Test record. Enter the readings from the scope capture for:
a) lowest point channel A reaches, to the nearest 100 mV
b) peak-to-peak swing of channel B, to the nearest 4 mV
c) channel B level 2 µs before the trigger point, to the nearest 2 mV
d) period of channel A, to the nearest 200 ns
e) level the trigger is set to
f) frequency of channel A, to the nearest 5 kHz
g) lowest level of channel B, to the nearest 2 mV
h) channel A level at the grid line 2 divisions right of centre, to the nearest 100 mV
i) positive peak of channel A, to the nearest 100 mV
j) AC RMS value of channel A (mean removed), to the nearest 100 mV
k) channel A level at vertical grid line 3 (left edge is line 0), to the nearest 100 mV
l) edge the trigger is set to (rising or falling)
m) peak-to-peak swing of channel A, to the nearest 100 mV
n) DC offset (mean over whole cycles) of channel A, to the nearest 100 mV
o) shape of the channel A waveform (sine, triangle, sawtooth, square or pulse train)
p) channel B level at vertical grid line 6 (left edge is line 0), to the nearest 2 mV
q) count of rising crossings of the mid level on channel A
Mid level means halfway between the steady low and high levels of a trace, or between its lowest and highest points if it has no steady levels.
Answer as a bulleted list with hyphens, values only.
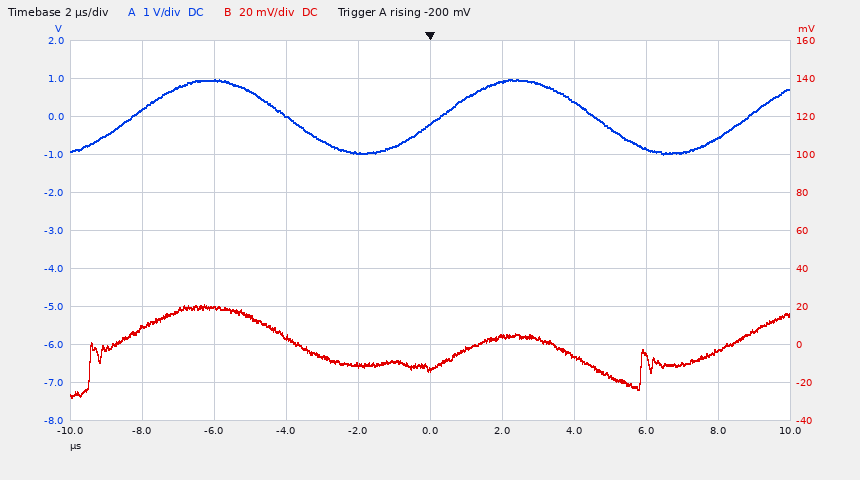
- -1.0 V
- 48 mV
- -10 mV
- 8.6 µs
- -200 mV
- 115 kHz
- -28 mV
- 400 mV
- 1.0 V
- 700 mV
- 0.0 V
- rising
- 2.0 V
- 0.0 V
- sine
- 4 mV
- 3
